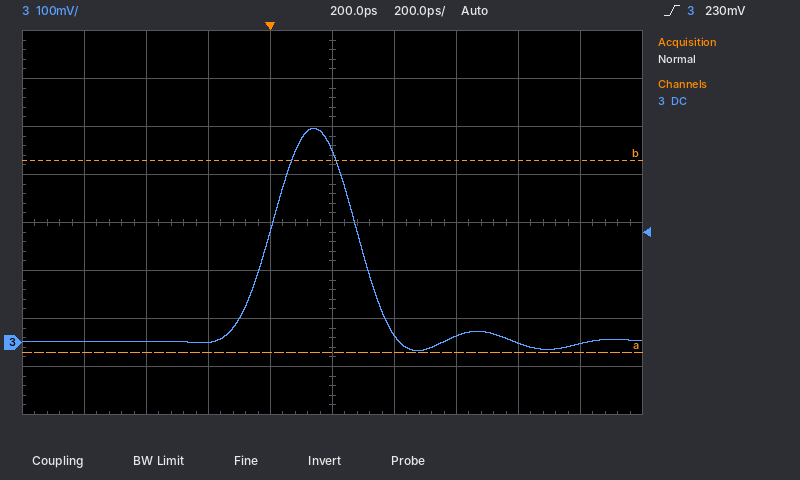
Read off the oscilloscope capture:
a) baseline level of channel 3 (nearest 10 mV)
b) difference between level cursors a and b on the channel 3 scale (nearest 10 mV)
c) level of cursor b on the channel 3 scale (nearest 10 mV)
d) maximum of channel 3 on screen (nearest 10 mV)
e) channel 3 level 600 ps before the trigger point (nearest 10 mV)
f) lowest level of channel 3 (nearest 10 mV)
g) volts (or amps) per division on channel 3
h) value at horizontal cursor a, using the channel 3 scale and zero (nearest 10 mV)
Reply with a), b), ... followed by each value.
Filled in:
a) 0 mV
b) 400 mV
c) 380 mV
d) 450 mV
e) 0 mV
f) -20 mV
g) 100 mV
h) -20 mV
